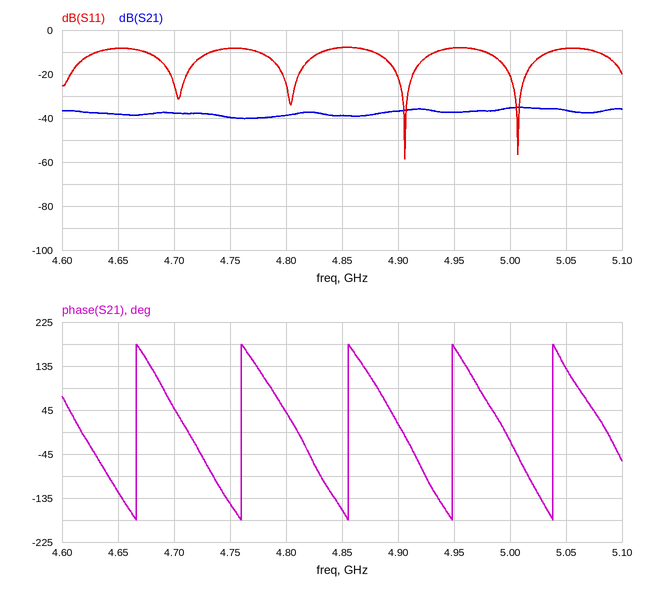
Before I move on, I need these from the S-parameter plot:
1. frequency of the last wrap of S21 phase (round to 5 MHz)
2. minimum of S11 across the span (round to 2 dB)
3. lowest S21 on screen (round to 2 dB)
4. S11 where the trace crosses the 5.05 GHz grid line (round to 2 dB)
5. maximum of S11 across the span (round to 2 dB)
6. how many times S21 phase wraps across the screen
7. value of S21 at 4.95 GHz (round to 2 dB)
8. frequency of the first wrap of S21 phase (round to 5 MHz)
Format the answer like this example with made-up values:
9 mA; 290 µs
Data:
5.040 GHz; -58 dB; -40 dB; -8 dB; -8 dB; 5; -38 dB; 4.665 GHz
